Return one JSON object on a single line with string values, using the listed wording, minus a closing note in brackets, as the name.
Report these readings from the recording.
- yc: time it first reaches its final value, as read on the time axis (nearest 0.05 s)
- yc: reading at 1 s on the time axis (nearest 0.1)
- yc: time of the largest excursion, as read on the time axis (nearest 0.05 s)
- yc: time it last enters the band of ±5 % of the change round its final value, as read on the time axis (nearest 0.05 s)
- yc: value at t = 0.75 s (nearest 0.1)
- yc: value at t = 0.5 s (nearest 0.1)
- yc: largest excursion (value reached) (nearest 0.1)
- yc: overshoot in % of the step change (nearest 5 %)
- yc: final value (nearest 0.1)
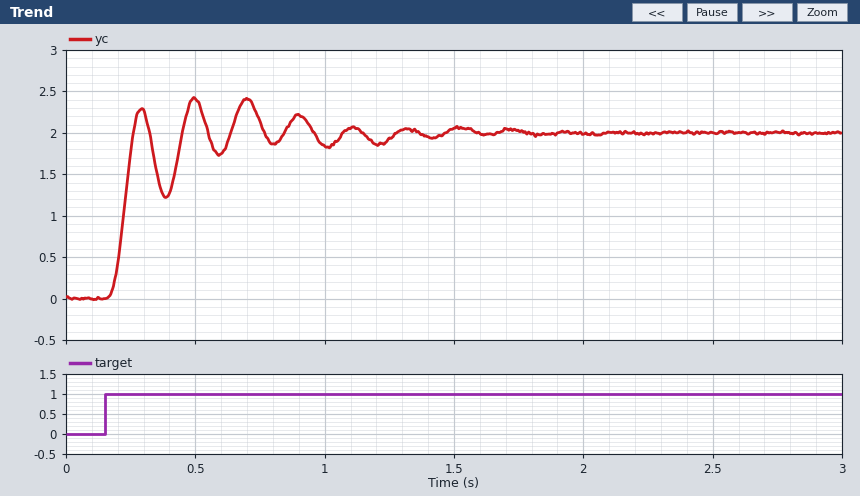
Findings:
{"yc: time it first reaches its final value, as read on the time axis": "0.25 s", "yc: reading at 1 s on the time axis": "1.8", "yc: time of the largest excursion, as read on the time axis": "0.50 s", "yc: time it last enters the band of ±5 % of the change round its final value, as read on the time axis": "1.25 s", "yc: value at t = 0.75 s": "2.1", "yc: value at t = 0.5 s": "2.4", "yc: largest excursion (value reached)": "2.4", "yc: overshoot in % of the step change": "20 %", "yc: final value": "2.0"}
